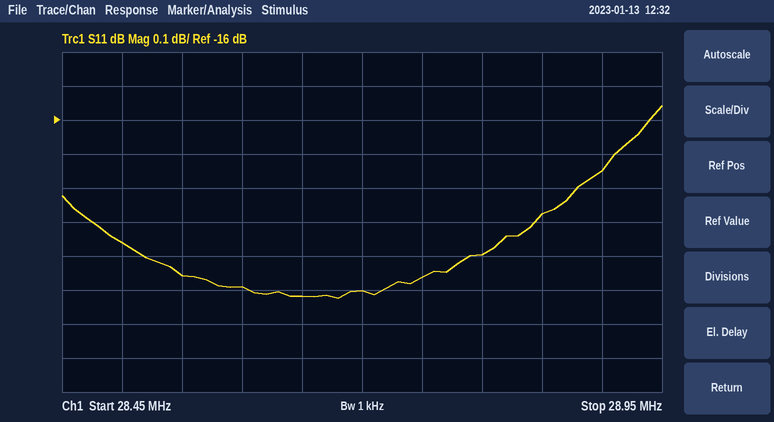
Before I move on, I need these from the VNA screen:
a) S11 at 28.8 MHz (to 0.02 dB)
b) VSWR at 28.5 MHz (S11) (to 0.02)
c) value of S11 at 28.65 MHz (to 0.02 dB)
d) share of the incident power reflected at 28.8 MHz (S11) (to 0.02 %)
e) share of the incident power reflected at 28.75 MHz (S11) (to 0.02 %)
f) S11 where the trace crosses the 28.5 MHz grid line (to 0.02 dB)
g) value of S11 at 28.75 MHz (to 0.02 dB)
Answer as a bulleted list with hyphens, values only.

- -16.40 dB
- 1.36
- -16.52 dB
- 2.30 %
- 2.26 %
- -16.36 dB
- -16.46 dB
